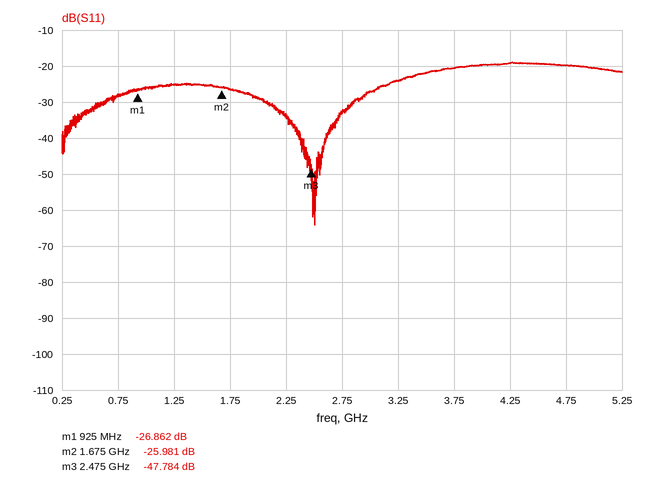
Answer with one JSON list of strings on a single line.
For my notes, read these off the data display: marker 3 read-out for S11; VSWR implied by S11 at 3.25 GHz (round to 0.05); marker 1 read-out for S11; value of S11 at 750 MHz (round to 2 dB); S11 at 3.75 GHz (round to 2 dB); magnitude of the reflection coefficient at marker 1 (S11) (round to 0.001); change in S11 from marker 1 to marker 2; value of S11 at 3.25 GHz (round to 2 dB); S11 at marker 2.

["-47.784 dB", "1.15", "-26.862 dB", "-28 dB", "-20 dB", "0.045", "0.881 dB", "-24 dB", "-25.981 dB"]
